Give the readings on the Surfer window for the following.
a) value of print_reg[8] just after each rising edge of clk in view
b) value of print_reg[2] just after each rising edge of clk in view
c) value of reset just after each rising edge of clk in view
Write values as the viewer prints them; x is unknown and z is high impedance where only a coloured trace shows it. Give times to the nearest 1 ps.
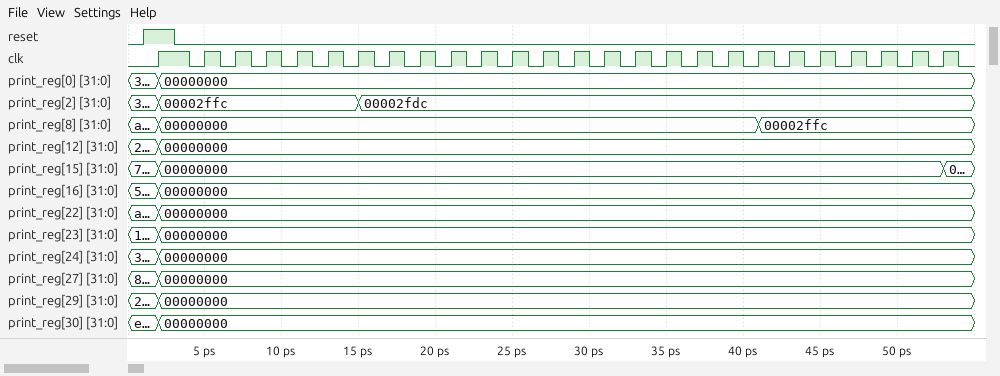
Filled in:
00000000, 00000000, 00000000, 00000000, 00000000, 00000000, 00000000, 00000000, 00000000, 00000000, 00000000, 00000000, 00000000, 00000000, 00000000, 00000000, 00000000, 00000000, 00000000, 00002ffc, 00002ffc, 00002ffc, 00002ffc, 00002ffc, 00002ffc, 00002ffc
00002ffc, 00002ffc, 00002ffc, 00002ffc, 00002ffc, 00002ffc, 00002fdc, 00002fdc, 00002fdc, 00002fdc, 00002fdc, 00002fdc, 00002fdc, 00002fdc, 00002fdc, 00002fdc, 00002fdc, 00002fdc, 00002fdc, 00002fdc, 00002fdc, 00002fdc, 00002fdc, 00002fdc, 00002fdc, 00002fdc
1 0 0 0 0 0 0 0 0 0 0 0 0 0 0 0 0 0 0 0 0 0 0 0 0 0
